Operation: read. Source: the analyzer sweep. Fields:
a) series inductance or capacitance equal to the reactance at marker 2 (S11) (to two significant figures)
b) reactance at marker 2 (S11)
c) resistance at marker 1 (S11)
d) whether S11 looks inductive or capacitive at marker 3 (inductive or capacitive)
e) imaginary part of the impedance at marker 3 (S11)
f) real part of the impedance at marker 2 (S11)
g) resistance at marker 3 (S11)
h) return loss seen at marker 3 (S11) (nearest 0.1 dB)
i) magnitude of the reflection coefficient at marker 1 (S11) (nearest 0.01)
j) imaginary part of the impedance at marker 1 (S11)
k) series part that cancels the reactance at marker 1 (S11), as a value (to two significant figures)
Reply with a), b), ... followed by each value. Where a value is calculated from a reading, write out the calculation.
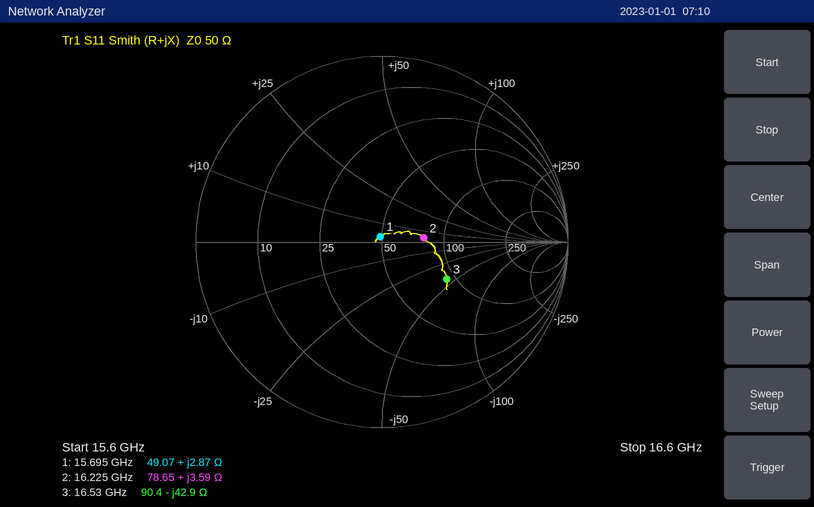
a) L = 3.59 Ω/(2π × 16.225 GHz) ≈ 35 pH
b) +3.59 Ω
c) 49.07 Ω
d) capacitive
e) -42.9 Ω
f) 78.65 Ω
g) 90.4 Ω
h) 7.9 dB
i) 0.03
j) +2.87 Ω
k) C = 1/(2π × 15.695 GHz × 2.87 Ω) ≈ 3.5 pF
